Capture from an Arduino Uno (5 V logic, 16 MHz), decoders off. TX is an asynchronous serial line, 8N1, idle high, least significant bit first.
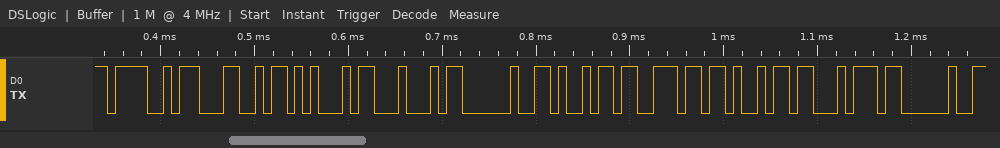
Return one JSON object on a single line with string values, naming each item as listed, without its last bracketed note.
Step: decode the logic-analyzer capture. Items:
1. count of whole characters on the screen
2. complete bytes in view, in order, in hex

{"count of whole characters on the screen": "10", "complete bytes in view, in order, in hex": "0x4F 0x4C 0x45 0x44 0x20 0x69 0x6E 0x69 0x74 0x20"}
